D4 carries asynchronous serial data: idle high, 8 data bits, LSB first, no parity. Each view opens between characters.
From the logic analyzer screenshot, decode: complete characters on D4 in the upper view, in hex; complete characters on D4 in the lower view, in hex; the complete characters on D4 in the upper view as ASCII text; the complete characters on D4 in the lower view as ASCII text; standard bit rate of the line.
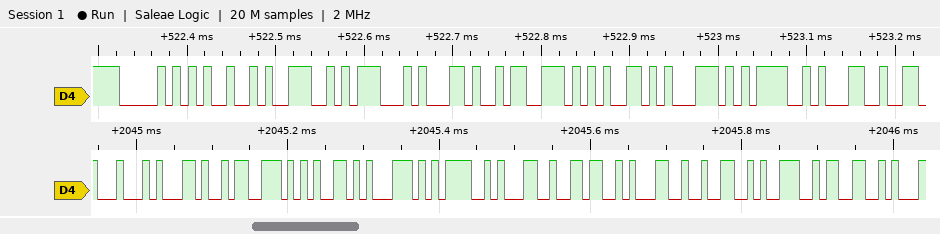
50, 49, 4E, 47, 2C, 73, 65, 71, 3D, 31
44, 2C, 73, 65, 71, 3D, 31, 36, 31, 32, 39, 33
"PING,seq=1"
"D,seq=161293"
115200 baud
